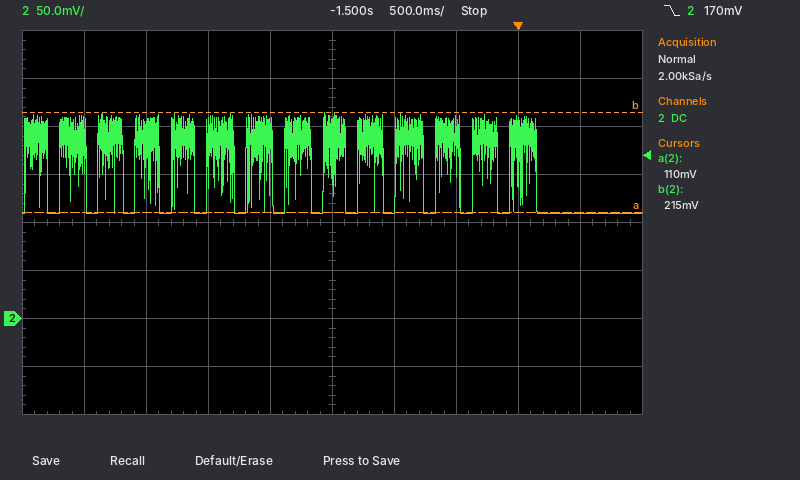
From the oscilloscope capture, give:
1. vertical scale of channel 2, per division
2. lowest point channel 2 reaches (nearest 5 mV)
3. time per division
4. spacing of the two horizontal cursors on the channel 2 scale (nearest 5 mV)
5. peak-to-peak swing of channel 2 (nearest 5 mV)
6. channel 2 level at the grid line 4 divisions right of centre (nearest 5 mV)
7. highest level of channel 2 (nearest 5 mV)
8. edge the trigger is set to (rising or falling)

50 mV
110 mV
500 ms
105 mV
105 mV
110 mV
215 mV
falling
